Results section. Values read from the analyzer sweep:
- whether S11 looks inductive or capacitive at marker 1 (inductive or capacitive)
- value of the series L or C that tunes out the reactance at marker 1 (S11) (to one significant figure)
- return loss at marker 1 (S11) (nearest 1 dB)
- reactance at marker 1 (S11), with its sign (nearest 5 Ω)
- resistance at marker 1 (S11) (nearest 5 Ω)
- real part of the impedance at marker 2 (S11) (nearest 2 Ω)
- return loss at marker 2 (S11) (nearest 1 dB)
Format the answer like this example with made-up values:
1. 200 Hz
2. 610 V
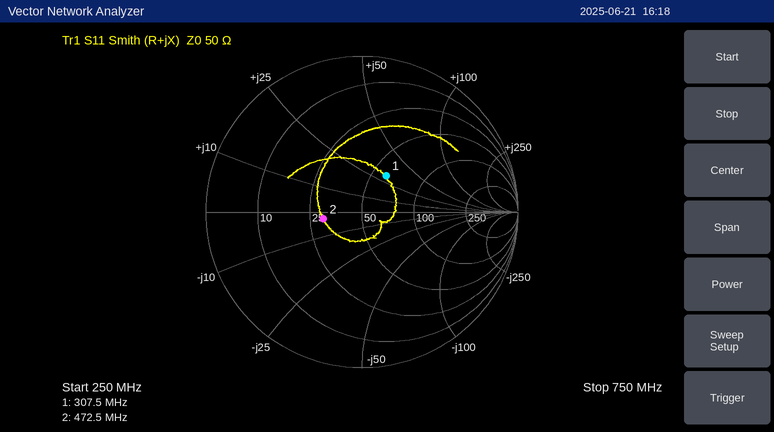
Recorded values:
1. inductive
2. 20 pF
3. 11 dB
4. +30 Ω
5. 60 Ω
6. 30 Ω
7. 12 dB
